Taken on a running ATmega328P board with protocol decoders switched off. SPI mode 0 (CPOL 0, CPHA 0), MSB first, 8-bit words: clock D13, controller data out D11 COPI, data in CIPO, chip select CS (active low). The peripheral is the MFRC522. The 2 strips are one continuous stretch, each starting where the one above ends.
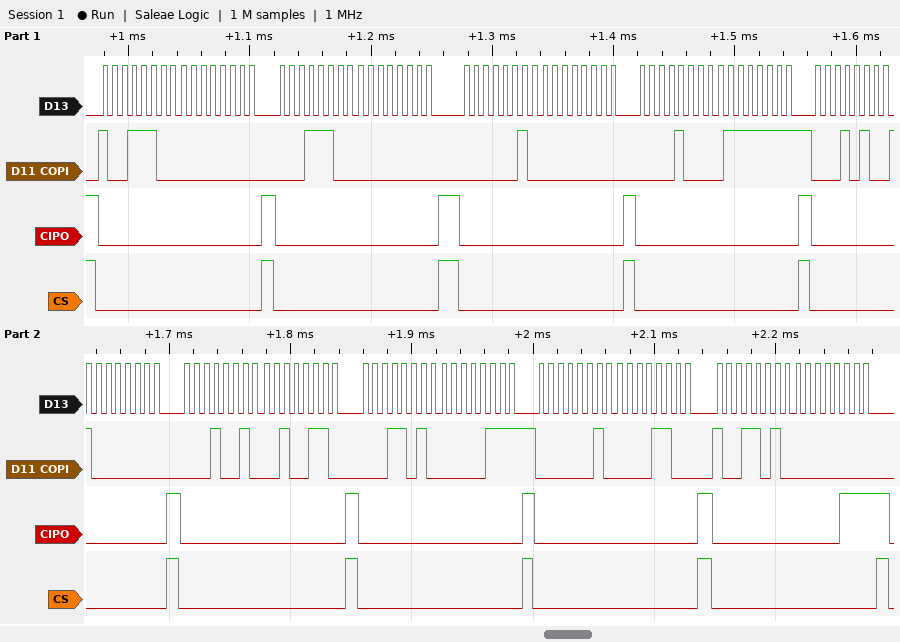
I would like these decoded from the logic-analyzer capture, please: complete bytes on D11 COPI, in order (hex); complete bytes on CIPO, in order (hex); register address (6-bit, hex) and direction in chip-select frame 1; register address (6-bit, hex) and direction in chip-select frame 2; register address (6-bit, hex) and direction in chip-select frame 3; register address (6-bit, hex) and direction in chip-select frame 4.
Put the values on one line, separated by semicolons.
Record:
0x9C 0x00 0x1C 0x00 0x02 0x00 0x08 0x7F 0x14 0x80 0x12 0x26 0x1A 0x07 0x02 0x0C 0x9A 0x00; 0x00 0x00 0x00 0x00 0x00 0x00 0x00 0x00 0x00 0x00 0x00 0x00 0x00 0x00 0x00 0x00 0x00 0x07; 0x0E read; 0x0E write; 0x01 write; 0x04 write
